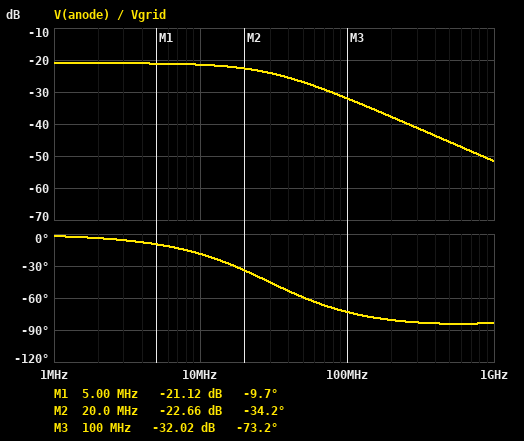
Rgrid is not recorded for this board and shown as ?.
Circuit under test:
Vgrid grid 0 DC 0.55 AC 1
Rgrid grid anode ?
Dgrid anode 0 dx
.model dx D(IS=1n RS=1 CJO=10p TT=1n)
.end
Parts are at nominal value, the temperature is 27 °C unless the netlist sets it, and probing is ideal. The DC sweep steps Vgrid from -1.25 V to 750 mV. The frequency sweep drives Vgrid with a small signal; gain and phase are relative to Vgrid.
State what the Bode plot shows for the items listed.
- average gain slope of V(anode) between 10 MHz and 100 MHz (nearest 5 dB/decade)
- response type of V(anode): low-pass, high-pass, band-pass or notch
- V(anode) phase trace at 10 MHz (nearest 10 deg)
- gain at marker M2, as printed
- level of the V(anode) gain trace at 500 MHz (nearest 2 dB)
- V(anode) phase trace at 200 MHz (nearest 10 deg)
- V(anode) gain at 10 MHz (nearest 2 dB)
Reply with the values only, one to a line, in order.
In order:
-10 dB/decade
low-pass
-20 deg
-22.66 dB
-46 dB
-80 deg
-22 dB
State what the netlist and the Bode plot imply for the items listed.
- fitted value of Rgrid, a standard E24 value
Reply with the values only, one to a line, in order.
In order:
4.3 kΩ
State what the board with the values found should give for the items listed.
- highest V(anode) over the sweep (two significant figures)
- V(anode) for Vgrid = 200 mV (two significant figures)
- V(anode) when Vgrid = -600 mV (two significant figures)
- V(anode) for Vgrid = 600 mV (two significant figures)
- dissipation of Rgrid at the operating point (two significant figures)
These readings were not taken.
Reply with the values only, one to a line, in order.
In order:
300 mV
190 mV
-600 mV
290 mV
16 µW
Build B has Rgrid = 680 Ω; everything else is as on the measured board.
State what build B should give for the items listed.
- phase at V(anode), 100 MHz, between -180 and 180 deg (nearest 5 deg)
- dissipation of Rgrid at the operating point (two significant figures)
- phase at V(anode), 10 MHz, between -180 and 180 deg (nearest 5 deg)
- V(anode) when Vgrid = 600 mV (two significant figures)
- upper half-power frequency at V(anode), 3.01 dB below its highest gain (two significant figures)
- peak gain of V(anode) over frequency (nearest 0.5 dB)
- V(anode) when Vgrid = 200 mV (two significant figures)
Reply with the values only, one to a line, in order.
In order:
-45 deg
72 µW
-5 deg
330 mV
90 MHz
-19.5 dB
200 mV
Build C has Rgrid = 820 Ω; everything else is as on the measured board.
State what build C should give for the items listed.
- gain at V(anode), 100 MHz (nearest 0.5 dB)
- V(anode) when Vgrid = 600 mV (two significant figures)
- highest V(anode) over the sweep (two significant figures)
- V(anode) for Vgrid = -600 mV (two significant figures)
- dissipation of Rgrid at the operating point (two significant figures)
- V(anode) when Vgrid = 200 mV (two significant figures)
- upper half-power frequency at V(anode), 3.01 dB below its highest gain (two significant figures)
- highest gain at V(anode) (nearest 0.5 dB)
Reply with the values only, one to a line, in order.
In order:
-23.5 dB
330 mV
340 mV
-600 mV
62 µW
200 mV
83 MHz
-19.5 dB
